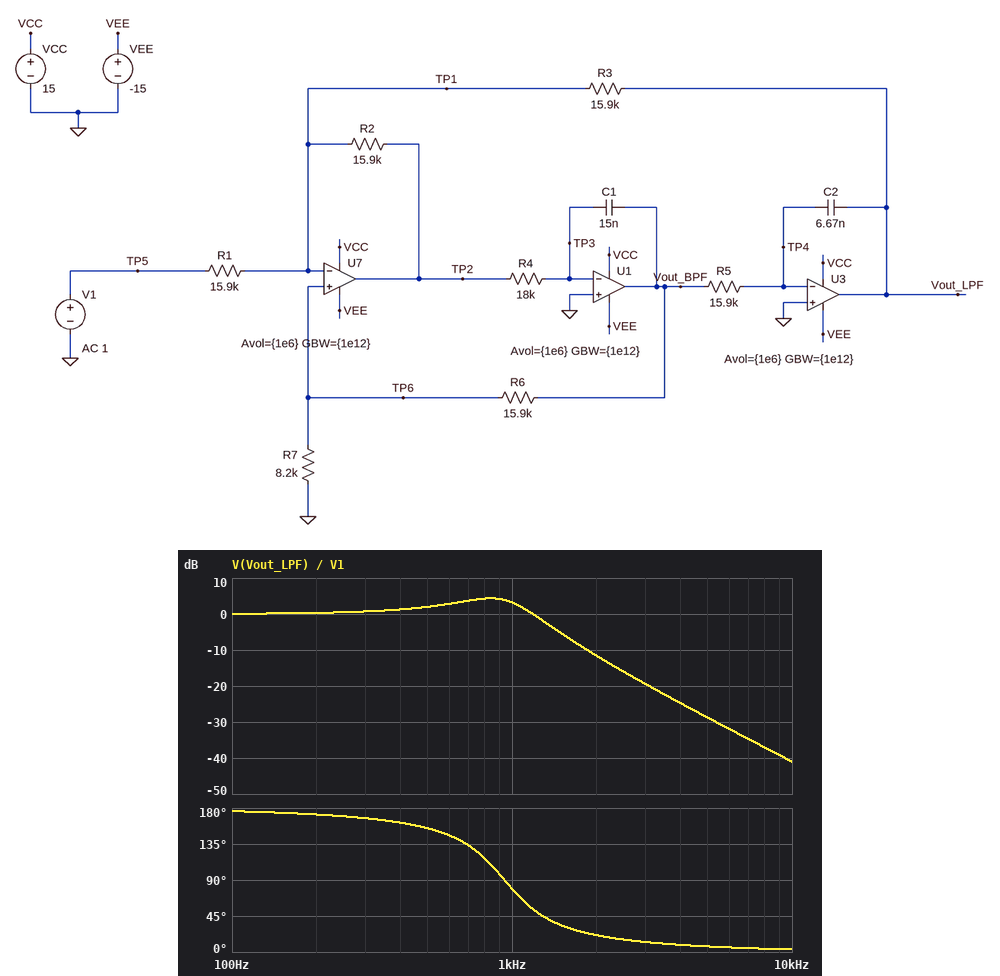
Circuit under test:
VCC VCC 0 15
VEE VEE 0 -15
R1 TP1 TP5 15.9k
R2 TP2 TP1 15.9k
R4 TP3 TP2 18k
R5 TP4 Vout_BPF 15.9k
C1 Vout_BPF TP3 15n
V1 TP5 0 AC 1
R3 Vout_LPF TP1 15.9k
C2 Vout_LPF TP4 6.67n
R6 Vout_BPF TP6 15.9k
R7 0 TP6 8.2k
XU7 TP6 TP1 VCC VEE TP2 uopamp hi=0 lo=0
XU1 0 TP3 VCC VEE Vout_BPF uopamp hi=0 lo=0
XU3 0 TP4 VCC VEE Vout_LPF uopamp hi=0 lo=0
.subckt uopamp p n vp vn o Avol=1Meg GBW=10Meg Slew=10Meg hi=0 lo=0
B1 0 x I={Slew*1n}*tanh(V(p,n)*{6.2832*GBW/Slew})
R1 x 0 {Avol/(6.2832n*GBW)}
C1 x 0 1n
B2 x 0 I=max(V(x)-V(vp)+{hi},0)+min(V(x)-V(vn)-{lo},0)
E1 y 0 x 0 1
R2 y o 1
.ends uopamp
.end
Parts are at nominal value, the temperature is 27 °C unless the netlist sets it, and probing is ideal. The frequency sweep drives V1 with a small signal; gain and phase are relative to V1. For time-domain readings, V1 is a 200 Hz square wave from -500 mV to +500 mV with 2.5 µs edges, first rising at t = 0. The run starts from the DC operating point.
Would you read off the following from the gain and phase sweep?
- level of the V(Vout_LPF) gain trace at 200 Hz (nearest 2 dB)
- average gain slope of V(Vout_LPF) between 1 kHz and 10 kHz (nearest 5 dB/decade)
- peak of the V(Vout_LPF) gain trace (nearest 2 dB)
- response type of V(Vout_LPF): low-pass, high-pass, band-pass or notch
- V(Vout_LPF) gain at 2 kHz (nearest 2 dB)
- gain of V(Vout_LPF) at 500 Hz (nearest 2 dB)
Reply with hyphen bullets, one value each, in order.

- 0 dB
- -45 dB/decade
- 4 dB
- low-pass
- -12 dB
- 2 dB
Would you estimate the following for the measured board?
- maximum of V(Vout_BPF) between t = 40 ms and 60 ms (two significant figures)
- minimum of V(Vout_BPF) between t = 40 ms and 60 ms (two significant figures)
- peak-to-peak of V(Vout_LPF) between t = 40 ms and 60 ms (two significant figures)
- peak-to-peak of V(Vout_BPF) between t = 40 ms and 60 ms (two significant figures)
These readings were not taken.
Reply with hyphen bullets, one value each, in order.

- 410 mV
- -410 mV
- 1.7 V
- 820 mV
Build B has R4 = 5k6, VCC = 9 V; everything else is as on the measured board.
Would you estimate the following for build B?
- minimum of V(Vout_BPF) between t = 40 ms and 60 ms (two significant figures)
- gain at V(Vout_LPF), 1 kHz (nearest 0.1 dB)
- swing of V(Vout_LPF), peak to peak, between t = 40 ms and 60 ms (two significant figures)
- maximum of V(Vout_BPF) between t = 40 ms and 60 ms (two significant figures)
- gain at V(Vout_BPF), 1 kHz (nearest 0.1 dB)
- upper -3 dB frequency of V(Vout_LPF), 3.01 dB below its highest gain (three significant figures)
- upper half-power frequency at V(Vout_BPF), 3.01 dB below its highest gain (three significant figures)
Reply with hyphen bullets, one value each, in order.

- -580 mV
- 0.5 dB
- 1.2 V
- 580 mV
- -3.0 dB
- 1.91 kHz
- 2.91 kHz
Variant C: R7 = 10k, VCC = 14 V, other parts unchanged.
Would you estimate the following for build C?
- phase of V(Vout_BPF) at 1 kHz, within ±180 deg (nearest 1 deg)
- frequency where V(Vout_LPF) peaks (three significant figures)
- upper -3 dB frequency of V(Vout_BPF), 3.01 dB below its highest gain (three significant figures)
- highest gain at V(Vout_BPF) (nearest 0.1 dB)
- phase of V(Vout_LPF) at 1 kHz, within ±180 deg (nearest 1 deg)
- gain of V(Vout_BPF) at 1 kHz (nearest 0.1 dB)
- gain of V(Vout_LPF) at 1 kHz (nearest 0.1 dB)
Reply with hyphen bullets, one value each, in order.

- -10 deg
- 807 Hz
- 1.34 kHz
- -1.3 dB
- 80 deg
- -1.4 dB
- 2.1 dB
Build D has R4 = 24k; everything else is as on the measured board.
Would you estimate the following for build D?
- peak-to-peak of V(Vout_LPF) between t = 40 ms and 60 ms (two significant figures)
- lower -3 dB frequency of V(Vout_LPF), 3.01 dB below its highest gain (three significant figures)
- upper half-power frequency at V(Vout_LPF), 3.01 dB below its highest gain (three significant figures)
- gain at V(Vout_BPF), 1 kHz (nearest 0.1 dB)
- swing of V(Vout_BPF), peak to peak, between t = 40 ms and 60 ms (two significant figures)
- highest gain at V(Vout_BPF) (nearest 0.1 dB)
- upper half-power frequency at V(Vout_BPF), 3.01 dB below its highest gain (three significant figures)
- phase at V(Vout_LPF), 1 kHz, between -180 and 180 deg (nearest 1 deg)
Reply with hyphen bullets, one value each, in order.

- 1.8 V
- 457 Hz
- 956 Hz
- -2.1 dB
- 730 mV
- -0.2 dB
- 1.07 kHz
- 53 deg
